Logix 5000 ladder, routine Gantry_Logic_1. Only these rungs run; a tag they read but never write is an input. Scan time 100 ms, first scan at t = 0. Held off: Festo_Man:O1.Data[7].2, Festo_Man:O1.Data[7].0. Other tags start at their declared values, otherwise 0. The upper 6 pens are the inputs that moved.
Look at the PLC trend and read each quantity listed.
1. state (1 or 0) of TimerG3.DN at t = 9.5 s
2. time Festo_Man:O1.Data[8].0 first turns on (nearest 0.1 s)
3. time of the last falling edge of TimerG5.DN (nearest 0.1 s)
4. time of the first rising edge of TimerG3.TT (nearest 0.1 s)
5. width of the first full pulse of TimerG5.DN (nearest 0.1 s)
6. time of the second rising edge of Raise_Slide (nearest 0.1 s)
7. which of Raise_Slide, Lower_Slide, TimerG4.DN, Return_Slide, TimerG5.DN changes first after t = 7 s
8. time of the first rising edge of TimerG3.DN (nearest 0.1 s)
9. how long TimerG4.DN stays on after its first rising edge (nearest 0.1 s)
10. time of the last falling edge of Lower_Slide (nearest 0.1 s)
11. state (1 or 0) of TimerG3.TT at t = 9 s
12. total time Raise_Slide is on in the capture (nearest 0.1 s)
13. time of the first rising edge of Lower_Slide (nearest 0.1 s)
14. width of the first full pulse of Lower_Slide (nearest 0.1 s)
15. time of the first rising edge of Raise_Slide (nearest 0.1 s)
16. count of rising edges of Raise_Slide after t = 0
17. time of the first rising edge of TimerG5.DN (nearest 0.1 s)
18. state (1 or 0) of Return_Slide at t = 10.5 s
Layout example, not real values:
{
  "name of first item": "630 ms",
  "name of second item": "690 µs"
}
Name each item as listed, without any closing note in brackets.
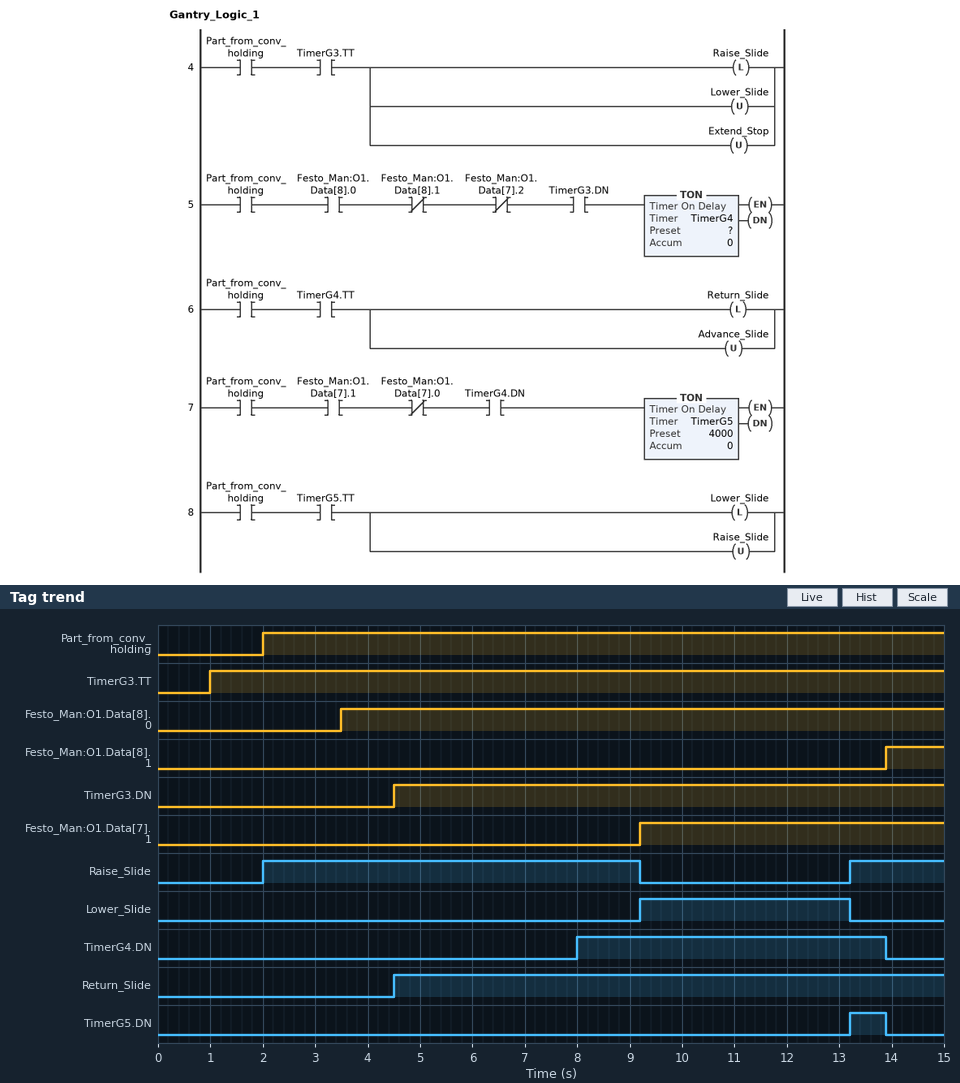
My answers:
{
  "state (1 or 0) of TimerG3.DN at t = 9.5 s": "1",
  "time Festo_Man:O1.Data[8].0 first turns on": "3.5 s",
  "time of the last falling edge of TimerG5.DN": "13.9 s",
  "time of the first rising edge of TimerG3.TT": "1.0 s",
  "width of the first full pulse of TimerG5.DN": "0.7 s",
  "time of the second rising edge of Raise_Slide": "13.2 s",
  "which of Raise_Slide, Lower_Slide, TimerG4.DN, Return_Slide, TimerG5.DN changes first after t = 7 s": "TimerG4.DN",
  "time of the first rising edge of TimerG3.DN": "4.5 s",
  "how long TimerG4.DN stays on after its first rising edge": "5.9 s",
  "time of the last falling edge of Lower_Slide": "13.2 s",
  "state (1 or 0) of TimerG3.TT at t = 9 s": "1",
  "total time Raise_Slide is on in the capture": "9.0 s",
  "time of the first rising edge of Lower_Slide": "9.2 s",
  "width of the first full pulse of Lower_Slide": "4.0 s",
  "time of the first rising edge of Raise_Slide": "2.0 s",
  "count of rising edges of Raise_Slide after t = 0": "2",
  "time of the first rising edge of TimerG5.DN": "13.2 s",
  "state (1 or 0) of Return_Slide at t = 10.5 s": "1"
}
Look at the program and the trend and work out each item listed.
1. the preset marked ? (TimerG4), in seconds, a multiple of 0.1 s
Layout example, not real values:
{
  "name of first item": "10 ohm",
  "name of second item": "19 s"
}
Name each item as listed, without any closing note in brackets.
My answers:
{
  "the preset marked ? (TimerG4), in seconds, a multiple of 0.1 s": "3.5 s"
}
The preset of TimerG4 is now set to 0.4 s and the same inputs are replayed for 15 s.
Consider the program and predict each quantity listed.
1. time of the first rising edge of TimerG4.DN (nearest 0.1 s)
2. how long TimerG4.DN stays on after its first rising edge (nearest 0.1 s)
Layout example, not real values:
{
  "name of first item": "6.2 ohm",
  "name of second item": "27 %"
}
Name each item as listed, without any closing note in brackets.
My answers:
{
  "time of the first rising edge of TimerG4.DN": "4.9 s",
  "how long TimerG4.DN stays on after its first rising edge": "9.0 s"
}
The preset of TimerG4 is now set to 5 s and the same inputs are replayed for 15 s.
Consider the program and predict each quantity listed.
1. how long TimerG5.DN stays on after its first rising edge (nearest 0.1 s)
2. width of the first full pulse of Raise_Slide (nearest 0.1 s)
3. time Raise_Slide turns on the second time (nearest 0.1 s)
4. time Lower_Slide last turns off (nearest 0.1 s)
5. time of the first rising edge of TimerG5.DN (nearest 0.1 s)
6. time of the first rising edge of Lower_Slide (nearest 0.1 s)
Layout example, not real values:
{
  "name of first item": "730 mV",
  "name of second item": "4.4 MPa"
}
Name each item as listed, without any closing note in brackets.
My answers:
{
  "how long TimerG5.DN stays on after its first rising edge": "0.4 s",
  "width of the first full pulse of Raise_Slide": "7.5 s",
  "time Raise_Slide turns on the second time": "13.5 s",
  "time Lower_Slide last turns off": "13.5 s",
  "time of the first rising edge of TimerG5.DN": "13.5 s",
  "time of the first rising edge of Lower_Slide": "9.5 s"
}
